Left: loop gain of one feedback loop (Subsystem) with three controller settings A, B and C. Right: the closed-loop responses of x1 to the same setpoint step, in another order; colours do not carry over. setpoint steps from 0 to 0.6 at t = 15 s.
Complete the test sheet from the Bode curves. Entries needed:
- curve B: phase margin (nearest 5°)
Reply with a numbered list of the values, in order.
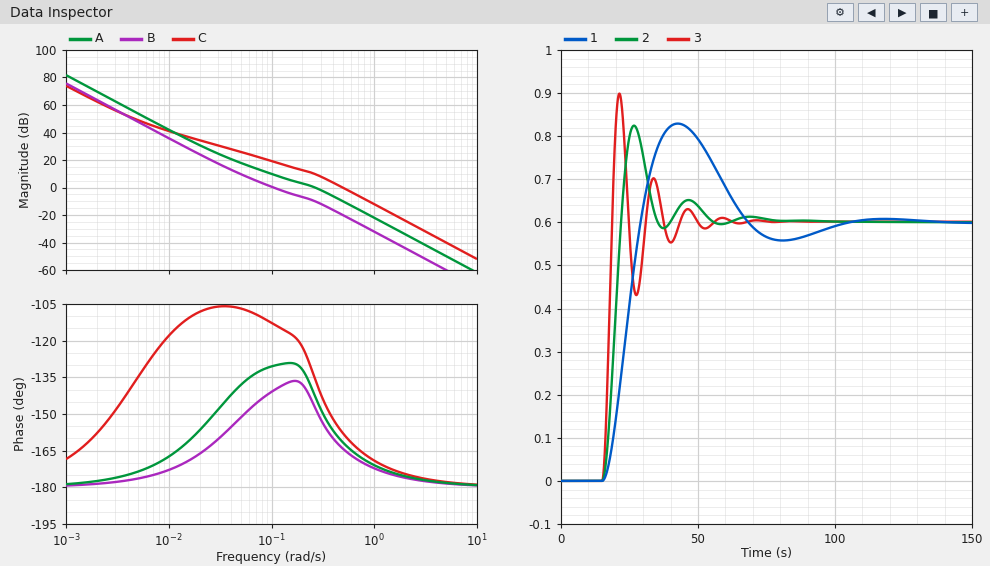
1. 40°
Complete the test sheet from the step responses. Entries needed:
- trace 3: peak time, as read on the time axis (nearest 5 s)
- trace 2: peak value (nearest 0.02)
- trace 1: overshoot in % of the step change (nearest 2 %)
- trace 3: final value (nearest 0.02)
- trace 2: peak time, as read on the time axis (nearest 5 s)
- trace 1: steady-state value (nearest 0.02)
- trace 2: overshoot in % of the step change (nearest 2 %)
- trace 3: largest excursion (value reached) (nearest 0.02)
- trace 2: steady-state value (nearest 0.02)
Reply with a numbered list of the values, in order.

1. 20 s
2. 0.82
3. 38 %
4. 0.60
5. 25 s
6. 0.60
7. 38 %
8. 0.90
9. 0.60
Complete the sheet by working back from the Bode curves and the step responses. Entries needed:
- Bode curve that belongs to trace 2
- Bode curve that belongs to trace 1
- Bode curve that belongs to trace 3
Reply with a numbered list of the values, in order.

1. A
2. B
3. C
